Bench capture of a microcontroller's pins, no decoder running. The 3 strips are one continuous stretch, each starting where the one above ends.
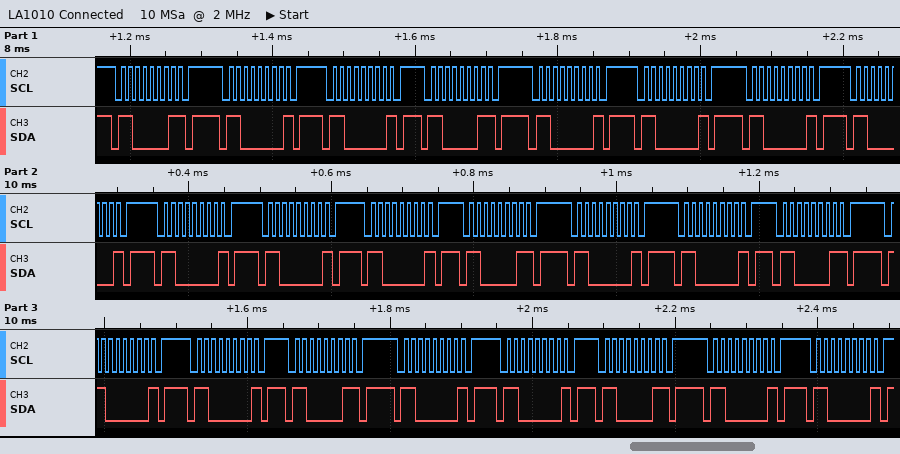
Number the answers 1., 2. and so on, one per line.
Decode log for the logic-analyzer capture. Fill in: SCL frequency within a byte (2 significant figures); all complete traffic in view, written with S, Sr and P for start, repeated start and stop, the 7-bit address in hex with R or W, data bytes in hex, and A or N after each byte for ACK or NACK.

1. 100 kHz
2. S 60R N P S 60W N P S 60W N P S 60R N P S 60W N P S 60W N P S 60W N P S 60W N P S 60W N P S 60W N P S 60W N P S 60R N P S 60W N P S 60W N P S 60R N P S 60W N P S 60W N P S 60R N P S 60W N P S 60W N P S 60R N P S 60W N P S 60W N P
